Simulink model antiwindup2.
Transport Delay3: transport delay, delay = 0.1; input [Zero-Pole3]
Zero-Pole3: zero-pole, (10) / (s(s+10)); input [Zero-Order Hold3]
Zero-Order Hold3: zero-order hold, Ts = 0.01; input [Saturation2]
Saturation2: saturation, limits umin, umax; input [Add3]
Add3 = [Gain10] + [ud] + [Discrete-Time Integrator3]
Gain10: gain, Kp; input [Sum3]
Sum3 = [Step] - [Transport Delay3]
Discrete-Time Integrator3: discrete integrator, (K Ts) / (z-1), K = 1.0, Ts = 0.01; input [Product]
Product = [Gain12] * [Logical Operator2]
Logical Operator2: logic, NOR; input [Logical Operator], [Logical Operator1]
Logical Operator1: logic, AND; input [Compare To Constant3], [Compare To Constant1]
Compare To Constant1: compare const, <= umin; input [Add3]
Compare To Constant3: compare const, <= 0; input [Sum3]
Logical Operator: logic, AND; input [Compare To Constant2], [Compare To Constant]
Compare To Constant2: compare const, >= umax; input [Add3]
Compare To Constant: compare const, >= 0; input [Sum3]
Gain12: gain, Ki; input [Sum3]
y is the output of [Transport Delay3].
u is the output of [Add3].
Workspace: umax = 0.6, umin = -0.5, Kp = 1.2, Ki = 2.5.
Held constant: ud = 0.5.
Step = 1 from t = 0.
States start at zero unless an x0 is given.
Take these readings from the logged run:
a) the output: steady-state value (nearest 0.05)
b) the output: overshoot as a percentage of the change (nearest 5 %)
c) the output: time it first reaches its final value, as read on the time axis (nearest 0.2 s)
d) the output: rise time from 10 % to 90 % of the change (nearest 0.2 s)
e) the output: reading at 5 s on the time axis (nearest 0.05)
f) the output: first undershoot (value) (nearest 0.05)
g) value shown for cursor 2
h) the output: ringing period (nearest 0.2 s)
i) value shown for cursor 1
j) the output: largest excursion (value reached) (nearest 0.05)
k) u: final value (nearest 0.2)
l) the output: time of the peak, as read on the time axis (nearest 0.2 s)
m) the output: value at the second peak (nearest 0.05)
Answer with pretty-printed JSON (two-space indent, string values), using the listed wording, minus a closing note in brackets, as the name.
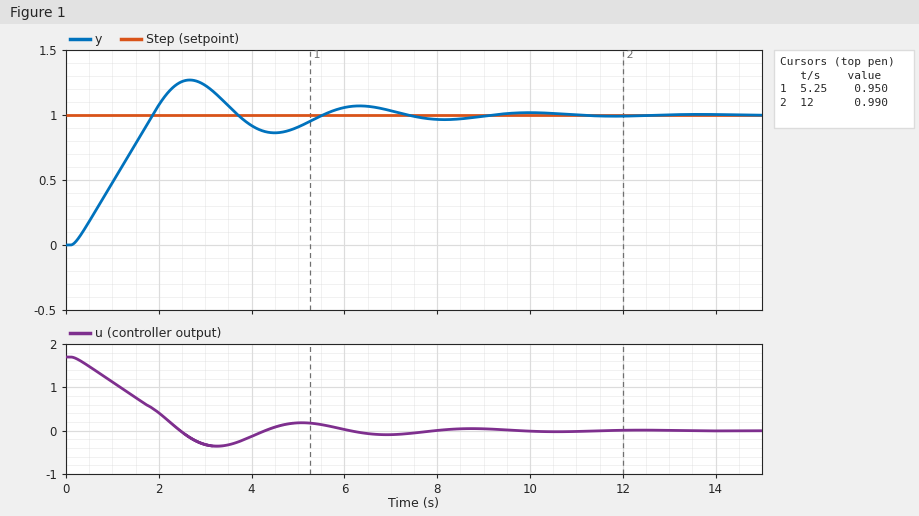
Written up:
{
  "the output: steady-state value": "1.00",
  "the output: overshoot as a percentage of the change": "25 %",
  "the output: time it first reaches its final value, as read on the time axis": "1.8 s",
  "the output: rise time from 10 % to 90 % of the change": "1.4 s",
  "the output: reading at 5 s on the time axis": "0.90",
  "the output: first undershoot (value)": "0.85",
  "value shown for cursor 2": "0.990",
  "the output: ringing period": "3.6 s",
  "value shown for cursor 1": "0.950",
  "the output: largest excursion (value reached)": "1.25",
  "u: final value": "0.0",
  "the output: time of the peak, as read on the time axis": "2.6 s",
  "the output: value at the second peak": "1.05"
}
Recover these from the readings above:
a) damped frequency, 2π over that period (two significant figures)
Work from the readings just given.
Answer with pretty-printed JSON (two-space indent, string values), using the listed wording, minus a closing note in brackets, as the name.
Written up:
{
  "damped frequency, 2π over that period": "1.7 rad/s"
}
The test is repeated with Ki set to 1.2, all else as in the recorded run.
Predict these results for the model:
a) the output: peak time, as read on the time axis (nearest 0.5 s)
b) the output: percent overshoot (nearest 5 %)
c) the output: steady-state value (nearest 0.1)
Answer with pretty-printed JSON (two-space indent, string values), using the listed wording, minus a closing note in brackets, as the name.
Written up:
{
  "the output: peak time, as read on the time axis": "3.0 s",
  "the output: percent overshoot": "30 %",
  "the output: steady-state value": "1.0"
}
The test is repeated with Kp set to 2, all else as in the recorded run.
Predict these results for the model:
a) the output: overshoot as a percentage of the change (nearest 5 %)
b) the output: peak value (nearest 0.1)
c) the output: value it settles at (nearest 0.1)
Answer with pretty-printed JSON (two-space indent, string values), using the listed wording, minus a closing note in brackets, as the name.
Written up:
{
  "the output: overshoot as a percentage of the change": "20 %",
  "the output: peak value": "1.2",
  "the output: value it settles at": "1.0"
}
